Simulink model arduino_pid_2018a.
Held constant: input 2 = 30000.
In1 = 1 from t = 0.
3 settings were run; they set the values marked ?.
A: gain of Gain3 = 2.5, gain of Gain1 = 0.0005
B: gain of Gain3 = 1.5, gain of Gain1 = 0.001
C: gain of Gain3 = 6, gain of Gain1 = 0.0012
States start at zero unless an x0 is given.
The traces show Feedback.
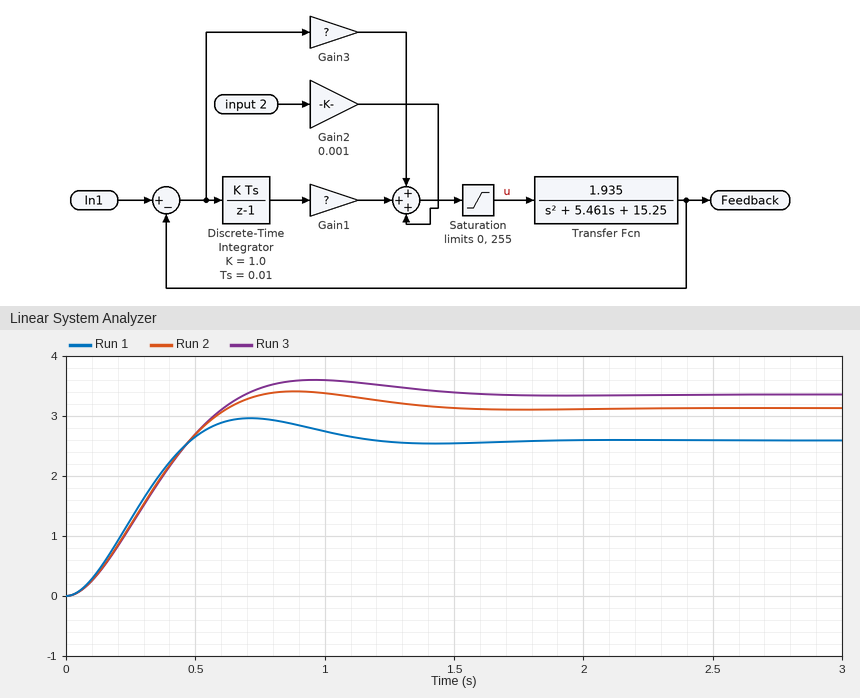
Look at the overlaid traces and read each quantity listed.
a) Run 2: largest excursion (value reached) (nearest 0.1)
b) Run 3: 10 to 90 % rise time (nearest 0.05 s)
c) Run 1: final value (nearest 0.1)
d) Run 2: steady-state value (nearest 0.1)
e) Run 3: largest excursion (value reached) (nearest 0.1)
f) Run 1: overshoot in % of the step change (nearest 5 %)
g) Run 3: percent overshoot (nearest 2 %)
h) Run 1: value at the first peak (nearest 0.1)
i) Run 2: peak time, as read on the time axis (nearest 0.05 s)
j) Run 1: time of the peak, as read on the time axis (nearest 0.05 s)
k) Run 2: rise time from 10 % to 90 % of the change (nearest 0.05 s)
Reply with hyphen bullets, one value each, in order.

- 3.4
- 0.45 s
- 2.6
- 3.1
- 3.6
- 15 %
- 8 %
- 3.0
- 0.90 s
- 0.70 s
- 0.40 s
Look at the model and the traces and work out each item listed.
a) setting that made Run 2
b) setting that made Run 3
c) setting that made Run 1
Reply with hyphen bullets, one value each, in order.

- A
- B
- C
